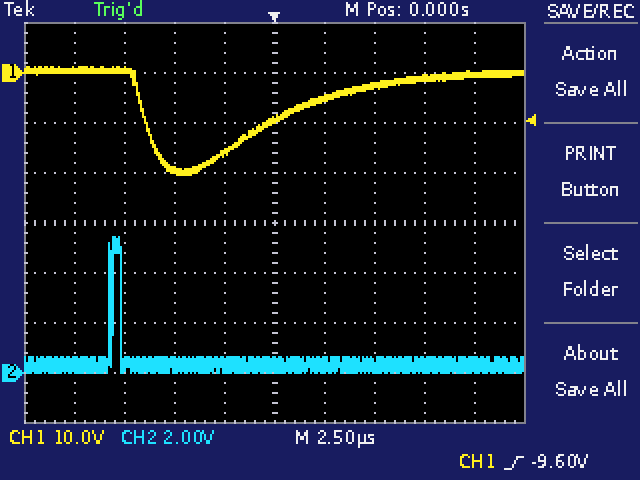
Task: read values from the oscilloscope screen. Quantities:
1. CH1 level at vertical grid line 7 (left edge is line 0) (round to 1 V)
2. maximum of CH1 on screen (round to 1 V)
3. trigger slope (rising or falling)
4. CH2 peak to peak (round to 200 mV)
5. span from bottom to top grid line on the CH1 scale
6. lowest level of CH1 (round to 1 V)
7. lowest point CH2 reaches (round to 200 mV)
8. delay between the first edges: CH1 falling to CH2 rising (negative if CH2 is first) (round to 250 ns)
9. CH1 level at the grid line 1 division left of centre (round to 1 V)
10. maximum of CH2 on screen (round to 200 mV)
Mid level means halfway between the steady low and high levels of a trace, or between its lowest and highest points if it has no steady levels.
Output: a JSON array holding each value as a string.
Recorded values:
["-3 V", "1 V", "rising", "5.4 V", "80 V", "-20 V", "0.0 V", "-1.75 µs", "-16 V", "5.4 V"]
